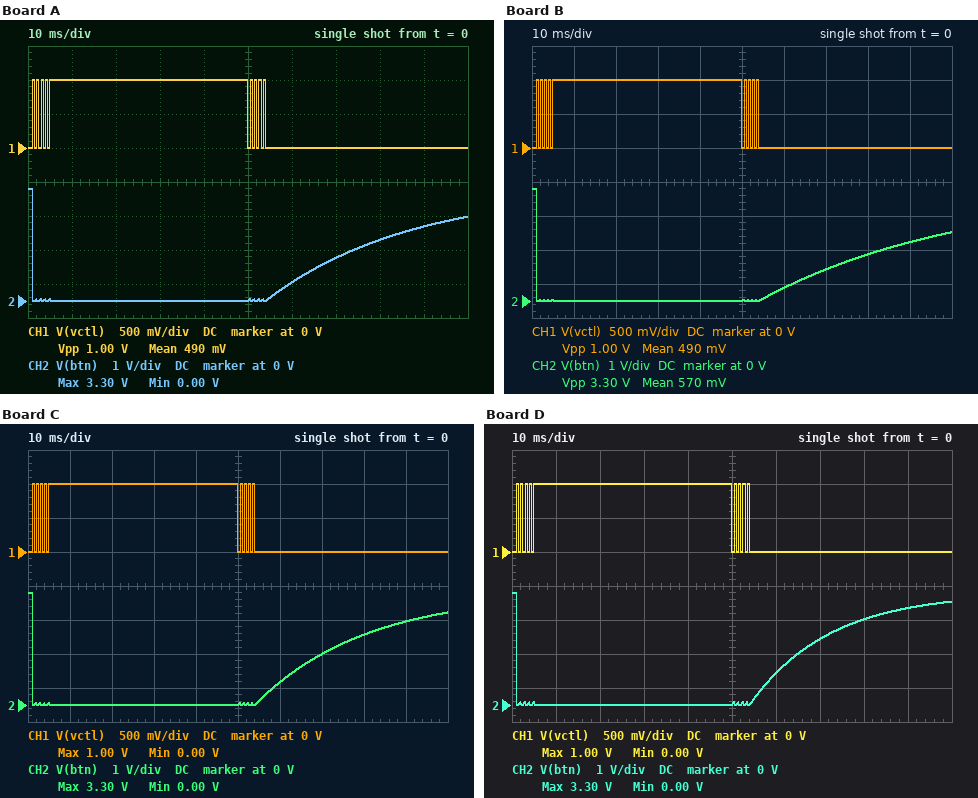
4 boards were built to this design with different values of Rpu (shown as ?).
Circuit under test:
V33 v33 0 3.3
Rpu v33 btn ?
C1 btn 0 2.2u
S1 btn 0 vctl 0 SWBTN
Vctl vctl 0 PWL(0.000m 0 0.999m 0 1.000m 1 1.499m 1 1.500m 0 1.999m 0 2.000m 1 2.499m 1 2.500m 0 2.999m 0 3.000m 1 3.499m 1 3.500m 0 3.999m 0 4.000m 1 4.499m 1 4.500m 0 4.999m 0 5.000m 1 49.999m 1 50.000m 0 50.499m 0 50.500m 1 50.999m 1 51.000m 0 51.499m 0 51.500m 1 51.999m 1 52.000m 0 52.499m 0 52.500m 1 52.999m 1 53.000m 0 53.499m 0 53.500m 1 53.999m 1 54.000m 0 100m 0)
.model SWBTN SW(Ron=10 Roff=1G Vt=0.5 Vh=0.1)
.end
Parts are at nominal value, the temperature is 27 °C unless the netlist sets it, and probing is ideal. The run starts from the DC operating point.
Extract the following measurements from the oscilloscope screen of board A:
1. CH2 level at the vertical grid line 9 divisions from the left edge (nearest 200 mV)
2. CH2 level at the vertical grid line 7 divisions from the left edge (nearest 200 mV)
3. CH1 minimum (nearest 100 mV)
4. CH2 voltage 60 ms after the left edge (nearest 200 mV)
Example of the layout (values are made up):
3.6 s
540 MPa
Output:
2.2 V
1.2 V
0 V
600 mV
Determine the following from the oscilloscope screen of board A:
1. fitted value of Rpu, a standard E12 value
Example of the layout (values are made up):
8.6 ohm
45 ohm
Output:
15 kΩ
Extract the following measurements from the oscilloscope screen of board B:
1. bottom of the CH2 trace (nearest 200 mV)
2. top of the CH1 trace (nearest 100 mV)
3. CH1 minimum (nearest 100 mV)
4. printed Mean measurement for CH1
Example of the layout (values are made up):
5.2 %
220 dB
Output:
0 V
1.0 V
0 V
490 mV
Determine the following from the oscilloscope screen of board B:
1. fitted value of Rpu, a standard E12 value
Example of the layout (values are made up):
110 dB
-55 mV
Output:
22 kΩ
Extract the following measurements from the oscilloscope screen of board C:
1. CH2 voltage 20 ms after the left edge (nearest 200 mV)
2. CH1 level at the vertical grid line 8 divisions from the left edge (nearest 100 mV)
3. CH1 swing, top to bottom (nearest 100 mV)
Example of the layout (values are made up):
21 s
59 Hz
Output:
0 V
0 V
1.0 V
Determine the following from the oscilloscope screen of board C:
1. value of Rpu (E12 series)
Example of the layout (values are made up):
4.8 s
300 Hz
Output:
12 kΩ
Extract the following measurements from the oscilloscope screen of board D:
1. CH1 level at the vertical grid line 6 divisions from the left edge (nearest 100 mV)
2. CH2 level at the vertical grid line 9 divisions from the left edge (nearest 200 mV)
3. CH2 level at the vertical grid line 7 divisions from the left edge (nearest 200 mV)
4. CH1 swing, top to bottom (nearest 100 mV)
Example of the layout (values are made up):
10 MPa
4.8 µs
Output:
0 V
2.8 V
2.0 V
1.0 V
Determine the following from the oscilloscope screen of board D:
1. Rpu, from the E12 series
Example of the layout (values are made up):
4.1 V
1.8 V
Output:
8.2 kΩ
